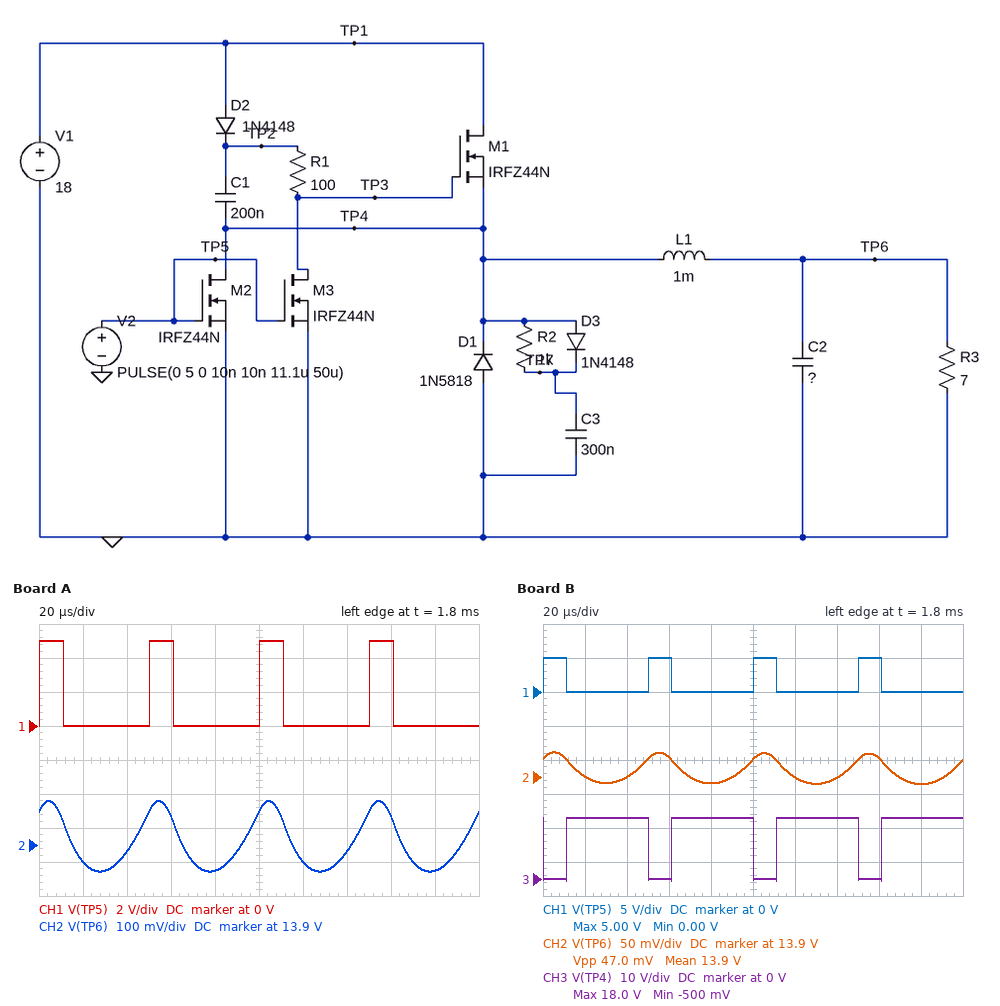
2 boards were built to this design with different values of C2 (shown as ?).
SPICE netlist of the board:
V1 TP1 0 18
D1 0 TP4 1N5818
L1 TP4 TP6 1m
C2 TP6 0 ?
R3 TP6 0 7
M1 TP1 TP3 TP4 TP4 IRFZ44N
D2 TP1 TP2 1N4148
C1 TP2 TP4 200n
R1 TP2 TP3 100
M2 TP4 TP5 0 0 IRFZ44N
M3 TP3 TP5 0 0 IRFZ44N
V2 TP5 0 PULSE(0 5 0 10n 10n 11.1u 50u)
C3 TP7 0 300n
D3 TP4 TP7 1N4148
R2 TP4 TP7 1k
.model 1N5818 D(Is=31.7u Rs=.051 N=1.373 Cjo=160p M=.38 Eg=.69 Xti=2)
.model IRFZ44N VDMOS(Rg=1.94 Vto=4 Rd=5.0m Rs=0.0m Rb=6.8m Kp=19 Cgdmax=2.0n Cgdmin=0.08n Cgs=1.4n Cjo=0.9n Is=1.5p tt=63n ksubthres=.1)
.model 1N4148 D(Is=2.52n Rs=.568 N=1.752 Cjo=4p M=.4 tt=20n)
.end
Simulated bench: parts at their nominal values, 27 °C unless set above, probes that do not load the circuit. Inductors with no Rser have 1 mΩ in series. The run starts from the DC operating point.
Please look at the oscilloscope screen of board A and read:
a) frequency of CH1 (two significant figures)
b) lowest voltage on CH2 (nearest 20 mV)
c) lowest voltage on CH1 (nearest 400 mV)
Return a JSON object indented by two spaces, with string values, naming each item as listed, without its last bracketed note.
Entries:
{
  "frequency of CH1": "20 kHz",
  "lowest voltage on CH2": "13.82 V",
  "lowest voltage on CH1": "0 V"
}
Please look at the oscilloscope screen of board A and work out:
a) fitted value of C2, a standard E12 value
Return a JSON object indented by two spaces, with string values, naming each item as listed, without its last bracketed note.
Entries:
{
  "fitted value of C2, a standard E12 value": "4.7 µF"
}
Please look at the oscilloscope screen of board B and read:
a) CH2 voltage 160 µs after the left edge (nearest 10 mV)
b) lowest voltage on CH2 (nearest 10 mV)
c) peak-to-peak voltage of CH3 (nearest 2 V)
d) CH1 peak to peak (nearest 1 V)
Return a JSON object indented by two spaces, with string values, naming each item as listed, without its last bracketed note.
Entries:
{
  "CH2 voltage 160 µs after the left edge": "13.93 V",
  "lowest voltage on CH2": "13.89 V",
  "peak-to-peak voltage of CH3": "18 V",
  "CH1 peak to peak": "5 V"
}
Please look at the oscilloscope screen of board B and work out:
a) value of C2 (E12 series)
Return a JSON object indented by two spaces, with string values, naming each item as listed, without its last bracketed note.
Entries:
{
  "value of C2": "22 µF"
}
